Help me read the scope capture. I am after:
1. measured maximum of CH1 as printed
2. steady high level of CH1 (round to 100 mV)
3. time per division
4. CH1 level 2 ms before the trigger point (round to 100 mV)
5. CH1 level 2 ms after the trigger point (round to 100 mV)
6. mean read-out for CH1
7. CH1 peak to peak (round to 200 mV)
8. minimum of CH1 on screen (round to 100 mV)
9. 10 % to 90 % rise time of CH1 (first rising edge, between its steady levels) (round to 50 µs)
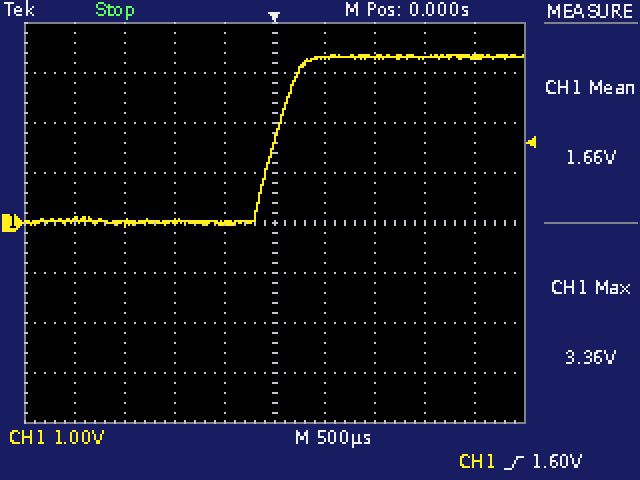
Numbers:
3.36 V
3.3 V
500 µs
100 mV
3.3 V
1.66 V
3.4 V
-100 mV
400 µs
